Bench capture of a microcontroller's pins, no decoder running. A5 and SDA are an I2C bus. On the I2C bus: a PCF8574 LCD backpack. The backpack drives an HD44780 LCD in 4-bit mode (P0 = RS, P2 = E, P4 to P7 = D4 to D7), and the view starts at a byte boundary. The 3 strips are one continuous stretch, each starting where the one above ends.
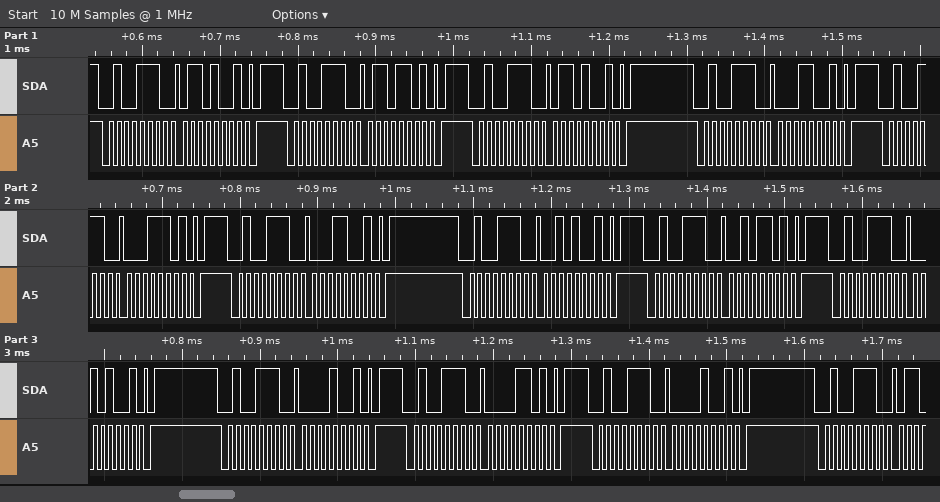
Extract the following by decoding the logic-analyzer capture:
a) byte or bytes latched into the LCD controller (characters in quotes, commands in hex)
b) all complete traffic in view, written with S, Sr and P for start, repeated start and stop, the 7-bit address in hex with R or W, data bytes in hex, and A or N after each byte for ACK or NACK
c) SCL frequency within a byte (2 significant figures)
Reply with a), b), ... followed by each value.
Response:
a) 'a' ' '
b) S 27W A 69 A P S 27W A 6D A P S 27W A 69 A P S 27W A 19 A P S 27W A 1D A P S 27W A 19 A P S 27W A 29 A P S 27W A 2D A P S 27W A 29 A P S 27W A 09 A P S 27W A 0D A P S 27W A 09 A P S 27W A
c) 100 kHz
